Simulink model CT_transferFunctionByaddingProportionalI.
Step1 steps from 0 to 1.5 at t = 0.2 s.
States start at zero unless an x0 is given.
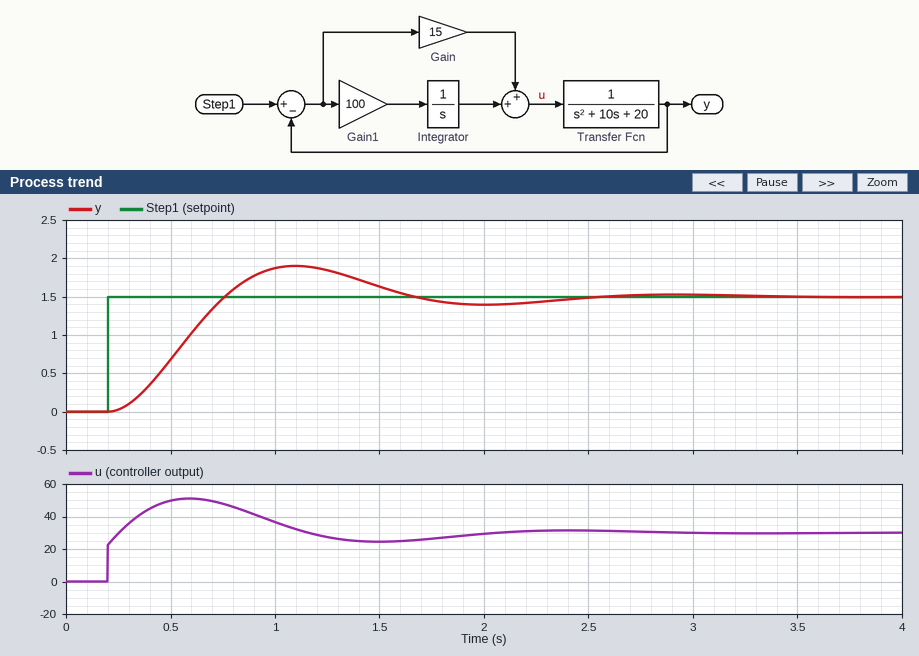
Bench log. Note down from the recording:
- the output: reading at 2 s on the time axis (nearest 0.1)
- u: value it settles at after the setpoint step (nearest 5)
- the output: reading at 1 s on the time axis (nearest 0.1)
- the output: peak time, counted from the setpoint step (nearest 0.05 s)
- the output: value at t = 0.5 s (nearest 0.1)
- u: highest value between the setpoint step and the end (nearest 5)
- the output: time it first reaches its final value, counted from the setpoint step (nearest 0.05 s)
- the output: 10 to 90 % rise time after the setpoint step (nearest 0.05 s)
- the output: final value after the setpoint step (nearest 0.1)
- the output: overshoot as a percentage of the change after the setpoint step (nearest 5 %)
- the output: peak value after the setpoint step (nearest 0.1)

1.4
30
1.9
0.90 s
0.7
50
0.55 s
0.40 s
1.5
25 %
1.9
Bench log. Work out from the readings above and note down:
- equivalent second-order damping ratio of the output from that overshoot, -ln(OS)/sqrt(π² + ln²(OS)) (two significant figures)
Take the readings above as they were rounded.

0.40
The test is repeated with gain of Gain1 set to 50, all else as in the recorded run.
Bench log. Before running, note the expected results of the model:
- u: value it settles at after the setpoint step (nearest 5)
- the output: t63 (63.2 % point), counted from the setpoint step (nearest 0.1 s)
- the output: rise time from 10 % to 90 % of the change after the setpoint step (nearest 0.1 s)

30
0.5 s
0.6 s
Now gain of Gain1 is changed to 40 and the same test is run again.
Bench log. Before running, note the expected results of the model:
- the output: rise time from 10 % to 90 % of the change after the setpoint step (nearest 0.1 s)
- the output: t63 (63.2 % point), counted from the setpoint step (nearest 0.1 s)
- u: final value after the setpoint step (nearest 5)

0.8 s
0.5 s
30
